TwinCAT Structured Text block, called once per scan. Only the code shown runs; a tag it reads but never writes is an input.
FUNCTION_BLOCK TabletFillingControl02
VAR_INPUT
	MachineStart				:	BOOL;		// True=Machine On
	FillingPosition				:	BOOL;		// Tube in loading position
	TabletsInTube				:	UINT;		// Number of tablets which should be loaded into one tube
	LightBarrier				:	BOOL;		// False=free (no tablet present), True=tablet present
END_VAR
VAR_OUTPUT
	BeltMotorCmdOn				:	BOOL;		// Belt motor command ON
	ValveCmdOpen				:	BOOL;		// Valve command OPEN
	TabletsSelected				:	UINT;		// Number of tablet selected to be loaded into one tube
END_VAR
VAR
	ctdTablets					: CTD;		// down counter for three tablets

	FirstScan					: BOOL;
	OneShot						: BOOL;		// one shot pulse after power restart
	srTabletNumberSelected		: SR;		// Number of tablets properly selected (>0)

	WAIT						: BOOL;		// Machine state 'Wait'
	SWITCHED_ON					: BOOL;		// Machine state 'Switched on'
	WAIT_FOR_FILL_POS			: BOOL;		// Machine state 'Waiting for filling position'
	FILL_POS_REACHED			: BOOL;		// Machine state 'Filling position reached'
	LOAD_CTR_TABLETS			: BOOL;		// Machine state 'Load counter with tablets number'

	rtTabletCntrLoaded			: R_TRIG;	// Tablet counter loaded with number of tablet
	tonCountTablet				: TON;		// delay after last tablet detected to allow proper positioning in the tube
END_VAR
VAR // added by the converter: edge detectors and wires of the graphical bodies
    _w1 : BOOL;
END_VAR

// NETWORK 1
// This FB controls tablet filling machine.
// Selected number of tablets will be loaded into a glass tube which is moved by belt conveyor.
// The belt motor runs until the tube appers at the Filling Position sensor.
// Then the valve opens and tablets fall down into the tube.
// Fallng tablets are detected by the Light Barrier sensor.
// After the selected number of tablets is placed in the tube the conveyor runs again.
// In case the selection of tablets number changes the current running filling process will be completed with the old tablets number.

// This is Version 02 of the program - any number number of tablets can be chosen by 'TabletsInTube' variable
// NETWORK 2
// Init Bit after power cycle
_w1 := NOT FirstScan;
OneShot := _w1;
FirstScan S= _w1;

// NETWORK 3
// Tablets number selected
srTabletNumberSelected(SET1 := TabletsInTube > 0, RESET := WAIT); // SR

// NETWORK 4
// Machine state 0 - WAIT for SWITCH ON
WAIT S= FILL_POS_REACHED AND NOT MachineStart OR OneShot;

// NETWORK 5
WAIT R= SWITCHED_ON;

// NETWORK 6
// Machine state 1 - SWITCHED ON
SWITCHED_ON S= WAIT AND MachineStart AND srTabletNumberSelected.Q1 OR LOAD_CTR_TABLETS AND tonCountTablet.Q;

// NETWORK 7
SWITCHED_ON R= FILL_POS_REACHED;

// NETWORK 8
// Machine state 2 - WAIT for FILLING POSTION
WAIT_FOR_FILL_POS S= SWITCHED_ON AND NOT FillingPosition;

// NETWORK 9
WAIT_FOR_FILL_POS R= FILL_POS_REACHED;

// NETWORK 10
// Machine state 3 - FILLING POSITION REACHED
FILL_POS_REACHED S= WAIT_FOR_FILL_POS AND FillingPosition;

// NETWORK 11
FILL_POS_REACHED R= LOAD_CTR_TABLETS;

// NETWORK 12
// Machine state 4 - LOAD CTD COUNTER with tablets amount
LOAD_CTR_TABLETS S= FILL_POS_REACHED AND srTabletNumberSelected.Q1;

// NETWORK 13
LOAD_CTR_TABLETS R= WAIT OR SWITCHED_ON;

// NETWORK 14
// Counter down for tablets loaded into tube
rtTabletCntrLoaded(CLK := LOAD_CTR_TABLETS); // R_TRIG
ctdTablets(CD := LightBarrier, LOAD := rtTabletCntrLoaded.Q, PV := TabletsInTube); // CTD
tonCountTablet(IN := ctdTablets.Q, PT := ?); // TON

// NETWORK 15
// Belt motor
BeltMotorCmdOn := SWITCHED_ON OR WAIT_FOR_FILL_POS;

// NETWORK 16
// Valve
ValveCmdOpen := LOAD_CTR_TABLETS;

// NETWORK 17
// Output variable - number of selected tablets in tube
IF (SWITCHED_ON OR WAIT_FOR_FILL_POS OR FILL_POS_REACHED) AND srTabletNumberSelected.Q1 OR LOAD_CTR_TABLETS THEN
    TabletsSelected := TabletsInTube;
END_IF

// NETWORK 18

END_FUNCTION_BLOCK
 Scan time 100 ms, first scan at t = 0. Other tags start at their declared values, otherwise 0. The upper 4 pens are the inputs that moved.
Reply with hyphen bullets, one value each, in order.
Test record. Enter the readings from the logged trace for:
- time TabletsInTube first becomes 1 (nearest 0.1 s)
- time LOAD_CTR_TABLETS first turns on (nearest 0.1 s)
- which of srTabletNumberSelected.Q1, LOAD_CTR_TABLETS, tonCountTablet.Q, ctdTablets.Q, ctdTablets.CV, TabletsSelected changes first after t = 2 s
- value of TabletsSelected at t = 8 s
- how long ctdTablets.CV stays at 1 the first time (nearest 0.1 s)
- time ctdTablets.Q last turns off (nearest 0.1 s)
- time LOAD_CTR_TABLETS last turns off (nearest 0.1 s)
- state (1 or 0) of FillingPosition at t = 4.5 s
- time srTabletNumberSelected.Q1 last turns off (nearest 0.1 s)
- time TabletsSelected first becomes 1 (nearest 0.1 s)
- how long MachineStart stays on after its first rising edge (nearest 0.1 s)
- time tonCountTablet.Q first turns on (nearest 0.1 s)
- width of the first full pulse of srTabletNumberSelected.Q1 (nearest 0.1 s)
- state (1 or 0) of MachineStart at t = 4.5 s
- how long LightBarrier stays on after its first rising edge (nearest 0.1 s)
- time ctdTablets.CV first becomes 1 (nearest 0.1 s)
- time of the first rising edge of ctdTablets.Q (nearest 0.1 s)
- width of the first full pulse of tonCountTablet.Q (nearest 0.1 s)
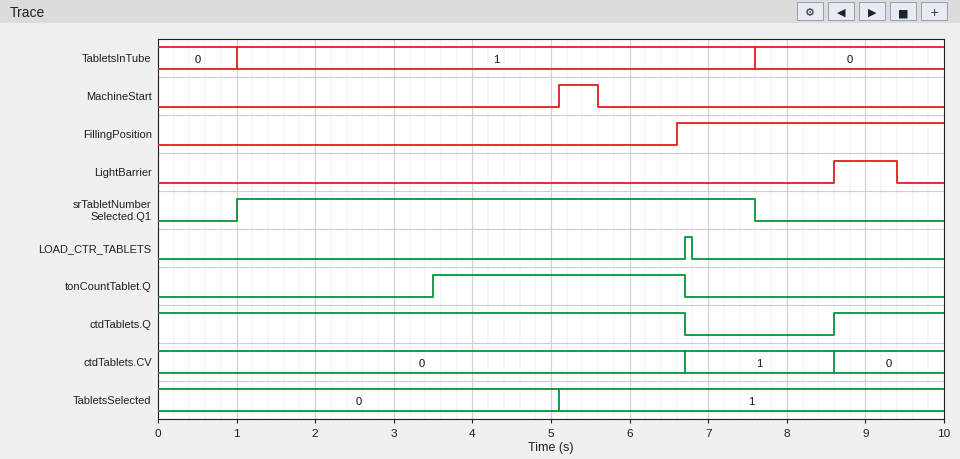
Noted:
- 1.0 s
- 6.7 s
- tonCountTablet.Q
- 1
- 1.9 s
- 6.7 s
- 6.8 s
- 0
- 7.6 s
- 5.1 s
- 0.5 s
- 3.5 s
- 6.6 s
- 0
- 0.8 s
- 6.7 s
- 8.6 s
- 3.2 s
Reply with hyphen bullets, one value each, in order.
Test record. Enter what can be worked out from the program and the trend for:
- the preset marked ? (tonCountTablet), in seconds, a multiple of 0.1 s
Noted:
- 3.5 s
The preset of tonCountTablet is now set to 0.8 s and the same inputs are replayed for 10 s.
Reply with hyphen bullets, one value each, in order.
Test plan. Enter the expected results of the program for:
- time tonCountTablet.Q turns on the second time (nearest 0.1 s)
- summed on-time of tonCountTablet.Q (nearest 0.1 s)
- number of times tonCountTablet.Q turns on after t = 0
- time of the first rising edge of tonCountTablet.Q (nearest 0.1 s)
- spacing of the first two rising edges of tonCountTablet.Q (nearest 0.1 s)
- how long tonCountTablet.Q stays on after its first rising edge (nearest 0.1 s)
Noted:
- 9.4 s
- 6.5 s
- 2
- 0.8 s
- 8.6 s
- 5.9 s
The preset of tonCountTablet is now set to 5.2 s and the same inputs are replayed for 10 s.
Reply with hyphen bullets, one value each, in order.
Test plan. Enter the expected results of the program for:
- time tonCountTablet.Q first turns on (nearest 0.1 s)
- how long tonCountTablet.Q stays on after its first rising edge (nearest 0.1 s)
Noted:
- 5.2 s
- 1.5 s
